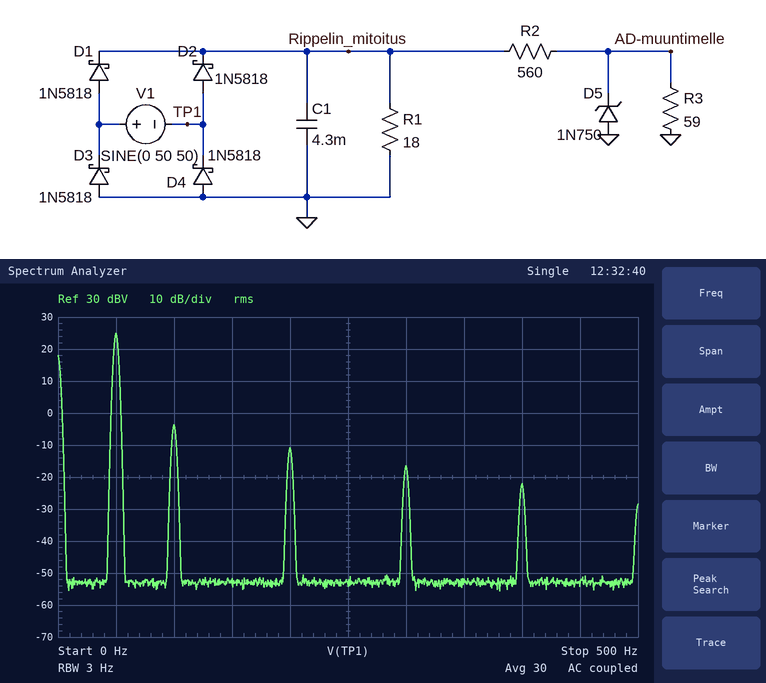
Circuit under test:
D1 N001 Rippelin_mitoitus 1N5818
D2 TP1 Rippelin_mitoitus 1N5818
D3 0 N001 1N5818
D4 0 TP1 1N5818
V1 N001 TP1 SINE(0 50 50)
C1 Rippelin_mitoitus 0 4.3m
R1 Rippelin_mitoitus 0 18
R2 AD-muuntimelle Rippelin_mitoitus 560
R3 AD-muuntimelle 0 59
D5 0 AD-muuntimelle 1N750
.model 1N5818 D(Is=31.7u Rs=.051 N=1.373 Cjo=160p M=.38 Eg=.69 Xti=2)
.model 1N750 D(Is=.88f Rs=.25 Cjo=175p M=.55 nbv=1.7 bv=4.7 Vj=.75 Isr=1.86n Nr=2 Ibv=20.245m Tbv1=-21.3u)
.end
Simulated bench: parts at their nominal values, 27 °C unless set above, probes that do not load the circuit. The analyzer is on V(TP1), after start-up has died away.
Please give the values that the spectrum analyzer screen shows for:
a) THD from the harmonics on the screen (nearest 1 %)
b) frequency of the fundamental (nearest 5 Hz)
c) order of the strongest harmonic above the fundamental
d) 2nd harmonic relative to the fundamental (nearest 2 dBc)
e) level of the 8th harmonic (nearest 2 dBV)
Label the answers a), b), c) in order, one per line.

a) 4 %
b) 50 Hz
c) 2
d) -28 dBc
e) -22 dBV
